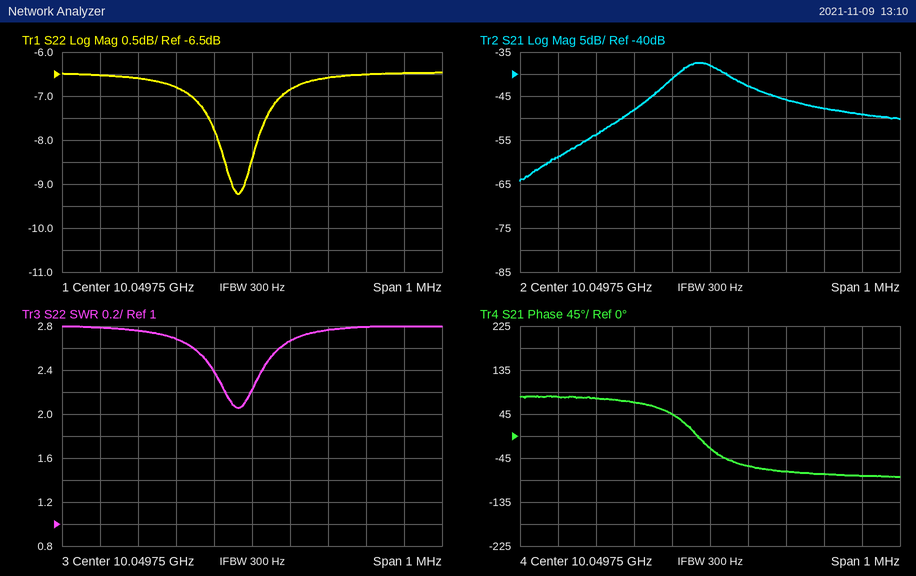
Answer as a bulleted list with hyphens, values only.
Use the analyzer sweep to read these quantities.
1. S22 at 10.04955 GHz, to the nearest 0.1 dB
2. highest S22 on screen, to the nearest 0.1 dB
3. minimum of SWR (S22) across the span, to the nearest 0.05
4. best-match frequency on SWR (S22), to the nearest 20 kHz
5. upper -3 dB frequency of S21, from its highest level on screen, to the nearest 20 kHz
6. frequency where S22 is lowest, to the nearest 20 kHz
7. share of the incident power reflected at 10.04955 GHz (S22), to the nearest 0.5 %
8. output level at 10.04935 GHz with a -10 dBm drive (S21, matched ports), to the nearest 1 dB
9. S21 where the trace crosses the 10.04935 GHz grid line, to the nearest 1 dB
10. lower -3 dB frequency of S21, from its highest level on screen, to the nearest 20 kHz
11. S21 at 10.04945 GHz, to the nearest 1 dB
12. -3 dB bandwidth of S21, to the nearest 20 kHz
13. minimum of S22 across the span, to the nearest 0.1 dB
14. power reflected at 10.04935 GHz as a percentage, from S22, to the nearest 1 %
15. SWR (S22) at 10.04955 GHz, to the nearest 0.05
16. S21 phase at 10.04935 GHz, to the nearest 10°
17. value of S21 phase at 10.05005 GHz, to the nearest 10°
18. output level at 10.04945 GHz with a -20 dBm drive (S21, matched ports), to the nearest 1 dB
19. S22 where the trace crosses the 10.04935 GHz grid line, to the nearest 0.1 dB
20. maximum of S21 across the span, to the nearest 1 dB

- -6.8 dB
- -6.5 dB
- 2.05
- 10.04972 GHz
- 10.04980 GHz
- 10.04972 GHz
- 21.0 %
- -69 dBm
- -59 dB
- 10.04966 GHz
- -54 dB
- 140 kHz
- -9.2 dB
- 22 %
- 2.70
- 80°
- -80°
- -74 dBm
- -6.5 dB
- -37 dB
